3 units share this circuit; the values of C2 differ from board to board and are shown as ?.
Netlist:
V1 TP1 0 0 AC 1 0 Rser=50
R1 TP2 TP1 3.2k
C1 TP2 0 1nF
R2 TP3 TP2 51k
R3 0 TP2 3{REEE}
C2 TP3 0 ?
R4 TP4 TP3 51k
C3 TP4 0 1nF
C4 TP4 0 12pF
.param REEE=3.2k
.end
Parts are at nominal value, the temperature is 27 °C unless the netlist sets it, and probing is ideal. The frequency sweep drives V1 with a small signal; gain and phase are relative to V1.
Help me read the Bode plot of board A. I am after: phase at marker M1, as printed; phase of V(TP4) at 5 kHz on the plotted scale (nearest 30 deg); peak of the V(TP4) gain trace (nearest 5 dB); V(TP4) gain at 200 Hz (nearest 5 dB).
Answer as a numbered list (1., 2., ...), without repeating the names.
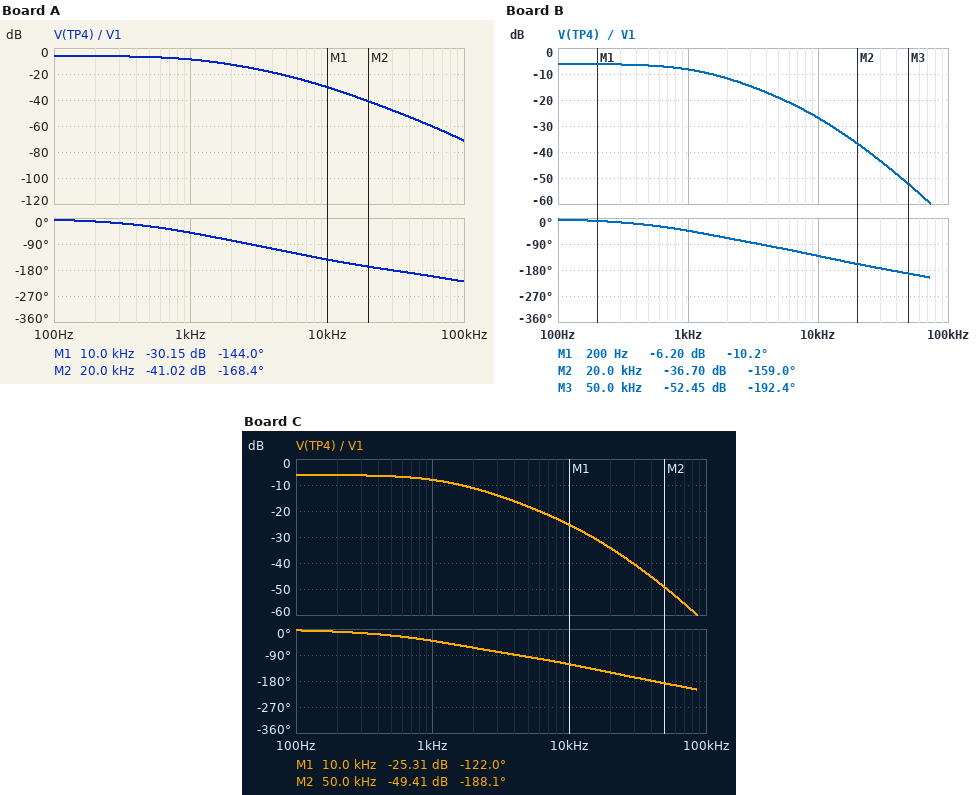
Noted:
1. -144.0 deg
2. -120 deg
3. -5 dB
4. -5 dB
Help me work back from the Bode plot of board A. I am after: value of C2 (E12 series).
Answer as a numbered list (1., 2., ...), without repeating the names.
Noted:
1. 1.2 nF
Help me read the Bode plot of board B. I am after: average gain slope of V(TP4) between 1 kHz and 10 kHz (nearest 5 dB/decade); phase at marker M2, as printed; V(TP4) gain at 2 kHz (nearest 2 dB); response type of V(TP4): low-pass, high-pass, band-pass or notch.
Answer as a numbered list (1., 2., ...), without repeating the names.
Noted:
1. -20 dB/decade
2. -159.0 deg
3. -12 dB
4. low-pass
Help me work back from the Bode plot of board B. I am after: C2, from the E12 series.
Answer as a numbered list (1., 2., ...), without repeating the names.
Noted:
1. 680 pF
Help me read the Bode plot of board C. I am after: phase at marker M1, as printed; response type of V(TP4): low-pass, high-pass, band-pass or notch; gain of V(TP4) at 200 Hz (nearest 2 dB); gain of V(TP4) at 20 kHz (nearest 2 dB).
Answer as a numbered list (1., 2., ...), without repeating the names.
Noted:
1. -122.0 deg
2. low-pass
3. -6 dB
4. -34 dB
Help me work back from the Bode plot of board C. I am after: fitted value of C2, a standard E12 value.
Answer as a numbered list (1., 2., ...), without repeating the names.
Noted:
1. 470 pF
